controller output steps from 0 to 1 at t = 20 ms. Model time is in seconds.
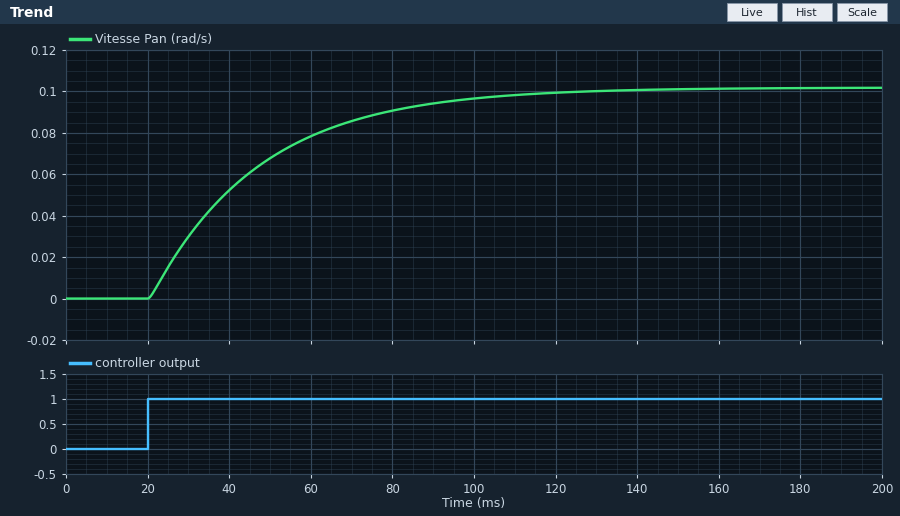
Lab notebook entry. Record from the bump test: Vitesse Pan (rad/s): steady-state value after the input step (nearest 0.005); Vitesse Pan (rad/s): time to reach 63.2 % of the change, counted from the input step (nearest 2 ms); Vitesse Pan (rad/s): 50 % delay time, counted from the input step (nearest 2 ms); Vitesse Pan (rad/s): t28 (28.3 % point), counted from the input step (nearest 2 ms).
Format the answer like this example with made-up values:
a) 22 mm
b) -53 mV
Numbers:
a) 0.100
b) 28 ms
c) 20 ms
d) 10 ms
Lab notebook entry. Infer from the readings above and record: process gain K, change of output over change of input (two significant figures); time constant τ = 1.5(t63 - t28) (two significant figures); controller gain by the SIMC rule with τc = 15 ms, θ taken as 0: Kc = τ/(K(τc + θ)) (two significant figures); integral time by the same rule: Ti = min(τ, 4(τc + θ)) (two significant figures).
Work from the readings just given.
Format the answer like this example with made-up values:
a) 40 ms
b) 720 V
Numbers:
a) 0.10
b) 27 ms
c) 18
d) 27 ms
